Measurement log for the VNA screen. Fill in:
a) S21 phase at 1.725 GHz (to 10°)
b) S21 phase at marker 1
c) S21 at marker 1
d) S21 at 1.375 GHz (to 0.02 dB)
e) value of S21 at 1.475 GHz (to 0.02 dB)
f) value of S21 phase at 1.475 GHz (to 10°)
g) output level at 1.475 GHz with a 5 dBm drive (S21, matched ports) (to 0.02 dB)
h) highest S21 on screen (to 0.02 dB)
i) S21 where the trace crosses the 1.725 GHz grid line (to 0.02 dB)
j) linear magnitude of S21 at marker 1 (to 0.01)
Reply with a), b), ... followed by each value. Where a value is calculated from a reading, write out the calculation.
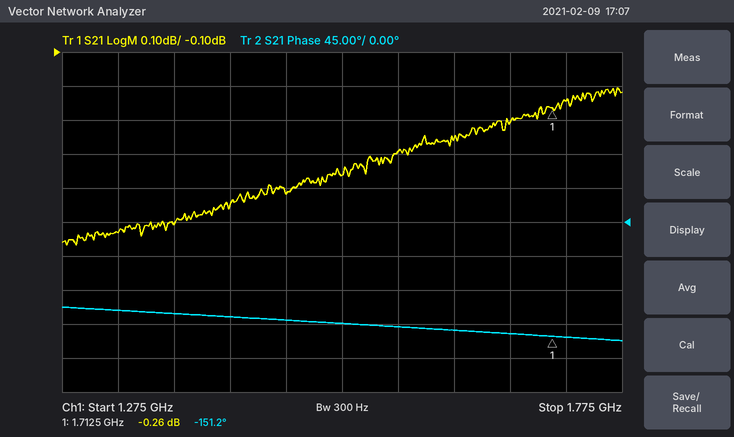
a) -150°
b) -151.2°
c) -0.26 dB
d) -0.60 dB
e) -0.52 dB
f) -130°
g) 5 dBm + (-0.52 dB) = 4.48 dBm
h) -0.20 dB
i) -0.24 dB
j) 10^(-0.26/20) ≈ 0.97
